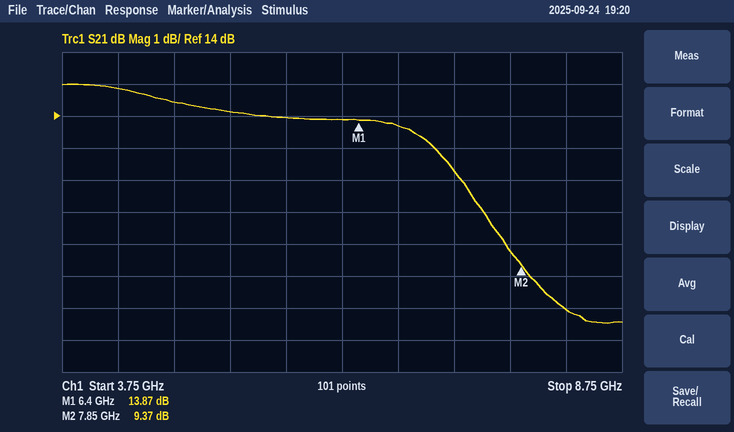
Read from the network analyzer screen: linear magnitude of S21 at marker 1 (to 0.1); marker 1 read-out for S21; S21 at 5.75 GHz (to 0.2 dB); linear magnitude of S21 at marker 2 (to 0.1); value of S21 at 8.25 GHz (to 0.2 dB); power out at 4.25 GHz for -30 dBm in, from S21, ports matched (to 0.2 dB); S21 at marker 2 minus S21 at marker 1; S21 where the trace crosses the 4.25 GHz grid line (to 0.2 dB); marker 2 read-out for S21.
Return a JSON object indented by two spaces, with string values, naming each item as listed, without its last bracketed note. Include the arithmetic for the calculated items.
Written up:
{
  "linear magnitude of S21 at marker 1": "10^(13.87/20) ≈ 4.9",
  "marker 1 read-out for S21": "13.87 dB",
  "S21 at 5.75 GHz": "14.0 dB",
  "linear magnitude of S21 at marker 2": "10^(9.37/20) ≈ 2.9",
  "value of S21 at 8.25 GHz": "8.0 dB",
  "power out at 4.25 GHz for -30 dBm in, from S21, ports matched": "-30 dBm + (14.8 dB) = -15.2 dBm",
  "S21 at marker 2 minus S21 at marker 1": "9.37 − (13.87) = -4.50 dB",
  "S21 where the trace crosses the 4.25 GHz grid line": "14.8 dB",
  "marker 2 read-out for S21": "9.37 dB"
}
